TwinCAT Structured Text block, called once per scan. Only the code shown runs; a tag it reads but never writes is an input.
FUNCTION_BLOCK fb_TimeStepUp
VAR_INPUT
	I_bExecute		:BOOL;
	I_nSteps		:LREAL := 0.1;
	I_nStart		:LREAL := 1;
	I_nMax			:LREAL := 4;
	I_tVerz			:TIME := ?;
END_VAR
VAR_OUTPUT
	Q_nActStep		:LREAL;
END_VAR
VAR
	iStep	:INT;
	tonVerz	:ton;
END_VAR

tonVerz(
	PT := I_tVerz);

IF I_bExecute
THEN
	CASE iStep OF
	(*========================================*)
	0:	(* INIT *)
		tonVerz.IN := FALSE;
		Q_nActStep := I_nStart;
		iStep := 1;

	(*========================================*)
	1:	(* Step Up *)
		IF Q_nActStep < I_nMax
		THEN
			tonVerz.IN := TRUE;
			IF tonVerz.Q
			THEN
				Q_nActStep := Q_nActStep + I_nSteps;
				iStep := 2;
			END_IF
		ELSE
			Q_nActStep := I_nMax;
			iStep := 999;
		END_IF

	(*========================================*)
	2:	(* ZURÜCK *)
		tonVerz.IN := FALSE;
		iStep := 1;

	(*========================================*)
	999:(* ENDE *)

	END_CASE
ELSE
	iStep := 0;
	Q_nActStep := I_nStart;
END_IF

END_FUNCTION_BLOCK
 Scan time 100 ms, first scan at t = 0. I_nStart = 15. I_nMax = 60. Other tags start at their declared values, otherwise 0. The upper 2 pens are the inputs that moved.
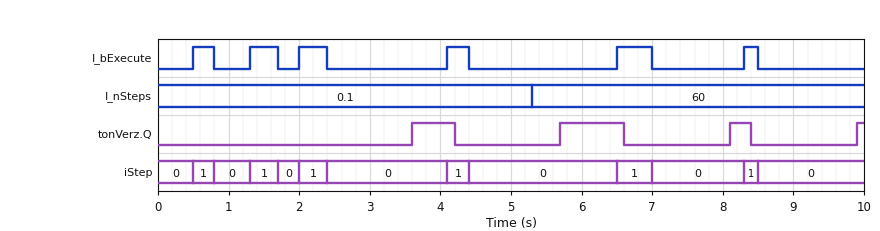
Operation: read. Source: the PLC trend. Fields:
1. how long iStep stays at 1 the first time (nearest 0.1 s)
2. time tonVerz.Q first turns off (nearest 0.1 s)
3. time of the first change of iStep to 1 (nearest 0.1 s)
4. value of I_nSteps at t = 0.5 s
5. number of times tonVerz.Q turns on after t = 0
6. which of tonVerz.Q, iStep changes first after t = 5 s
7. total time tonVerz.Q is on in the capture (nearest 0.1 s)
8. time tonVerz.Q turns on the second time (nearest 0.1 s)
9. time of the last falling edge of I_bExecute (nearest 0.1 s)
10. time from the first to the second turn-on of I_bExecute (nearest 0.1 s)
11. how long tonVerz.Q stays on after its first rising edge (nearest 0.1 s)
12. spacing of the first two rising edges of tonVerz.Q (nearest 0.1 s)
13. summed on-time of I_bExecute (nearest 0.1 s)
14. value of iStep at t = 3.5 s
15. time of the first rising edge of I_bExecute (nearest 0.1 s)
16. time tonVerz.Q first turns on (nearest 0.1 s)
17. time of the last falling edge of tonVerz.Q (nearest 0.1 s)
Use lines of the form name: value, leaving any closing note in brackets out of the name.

how long iStep stays at 1 the first time: 0.3 s
time tonVerz.Q first turns off: 4.2 s
time of the first change of iStep to 1: 0.5 s
value of I_nSteps at t = 0.5 s: 0.1
number of times tonVerz.Q turns on after t = 0: 4
which of tonVerz.Q, iStep changes first after t = 5 s: tonVerz.Q
total time tonVerz.Q is on in the capture: 1.9 s
time tonVerz.Q turns on the second time: 5.7 s
time of the last falling edge of I_bExecute: 8.5 s
time from the first to the second turn-on of I_bExecute: 0.8 s
how long tonVerz.Q stays on after its first rising edge: 0.6 s
spacing of the first two rising edges of tonVerz.Q: 2.1 s
summed on-time of I_bExecute: 2.1 s
value of iStep at t = 3.5 s: 0
time of the first rising edge of I_bExecute: 0.5 s
time tonVerz.Q first turns on: 3.6 s
time of the last falling edge of tonVerz.Q: 8.4 s
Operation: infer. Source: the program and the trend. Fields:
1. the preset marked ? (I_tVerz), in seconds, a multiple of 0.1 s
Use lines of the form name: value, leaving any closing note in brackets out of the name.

the preset marked ? (I_tVerz), in seconds, a multiple of 0.1 s: 1.4 s
